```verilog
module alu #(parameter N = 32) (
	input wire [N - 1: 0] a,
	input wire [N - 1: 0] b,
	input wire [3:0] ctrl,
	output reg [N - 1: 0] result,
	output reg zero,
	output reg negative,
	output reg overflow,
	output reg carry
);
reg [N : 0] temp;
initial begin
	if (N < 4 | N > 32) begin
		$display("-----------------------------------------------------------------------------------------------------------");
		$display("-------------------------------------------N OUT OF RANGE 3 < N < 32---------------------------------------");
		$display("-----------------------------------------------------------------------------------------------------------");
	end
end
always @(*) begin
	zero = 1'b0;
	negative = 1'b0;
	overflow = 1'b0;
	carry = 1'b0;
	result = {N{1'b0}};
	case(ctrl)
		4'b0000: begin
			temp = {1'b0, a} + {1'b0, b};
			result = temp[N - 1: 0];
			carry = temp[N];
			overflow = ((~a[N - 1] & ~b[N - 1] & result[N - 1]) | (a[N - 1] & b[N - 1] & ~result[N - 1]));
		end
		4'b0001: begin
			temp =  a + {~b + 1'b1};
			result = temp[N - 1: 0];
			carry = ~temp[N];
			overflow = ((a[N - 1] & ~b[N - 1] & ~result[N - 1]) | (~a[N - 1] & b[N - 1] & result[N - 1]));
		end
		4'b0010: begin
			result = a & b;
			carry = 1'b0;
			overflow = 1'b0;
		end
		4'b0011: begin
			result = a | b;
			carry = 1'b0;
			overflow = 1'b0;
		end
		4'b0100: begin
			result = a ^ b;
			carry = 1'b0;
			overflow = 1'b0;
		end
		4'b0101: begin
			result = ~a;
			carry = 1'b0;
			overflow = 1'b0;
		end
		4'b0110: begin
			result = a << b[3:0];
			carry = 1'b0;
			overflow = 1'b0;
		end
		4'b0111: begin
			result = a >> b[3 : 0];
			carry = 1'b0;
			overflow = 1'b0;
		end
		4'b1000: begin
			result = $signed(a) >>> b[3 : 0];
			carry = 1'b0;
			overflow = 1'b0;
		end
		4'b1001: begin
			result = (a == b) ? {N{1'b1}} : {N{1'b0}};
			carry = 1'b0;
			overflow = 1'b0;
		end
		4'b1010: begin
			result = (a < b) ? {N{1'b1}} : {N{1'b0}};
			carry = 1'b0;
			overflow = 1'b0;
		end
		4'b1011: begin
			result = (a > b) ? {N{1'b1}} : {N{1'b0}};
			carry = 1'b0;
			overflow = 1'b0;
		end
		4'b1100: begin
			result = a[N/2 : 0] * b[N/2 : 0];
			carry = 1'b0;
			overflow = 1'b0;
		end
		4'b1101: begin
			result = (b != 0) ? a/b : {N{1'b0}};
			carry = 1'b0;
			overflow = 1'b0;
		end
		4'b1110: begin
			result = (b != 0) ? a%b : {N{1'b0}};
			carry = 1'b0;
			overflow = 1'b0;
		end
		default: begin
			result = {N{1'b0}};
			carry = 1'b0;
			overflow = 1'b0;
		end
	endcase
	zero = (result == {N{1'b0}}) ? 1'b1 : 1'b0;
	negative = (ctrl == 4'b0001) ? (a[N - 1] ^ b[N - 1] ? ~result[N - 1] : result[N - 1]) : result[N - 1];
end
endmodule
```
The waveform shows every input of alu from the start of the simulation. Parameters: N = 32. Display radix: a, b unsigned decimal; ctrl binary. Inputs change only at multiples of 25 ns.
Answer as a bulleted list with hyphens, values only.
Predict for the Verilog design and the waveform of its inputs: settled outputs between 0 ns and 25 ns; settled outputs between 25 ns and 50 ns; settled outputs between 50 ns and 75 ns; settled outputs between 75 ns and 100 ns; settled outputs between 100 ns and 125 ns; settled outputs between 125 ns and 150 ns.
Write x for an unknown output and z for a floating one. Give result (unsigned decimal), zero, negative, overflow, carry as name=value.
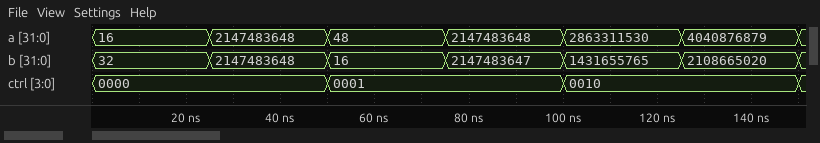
- result=48, zero=0, negative=0, overflow=0, carry=0
- result=0, zero=1, negative=0, overflow=1, carry=1
- result=32, zero=0, negative=0, overflow=0, carry=0
- result=1, zero=0, negative=1, overflow=1, carry=0
- result=0, zero=1, negative=0, overflow=0, carry=0
- result=1888133132, zero=0, negative=0, overflow=0, carry=0
